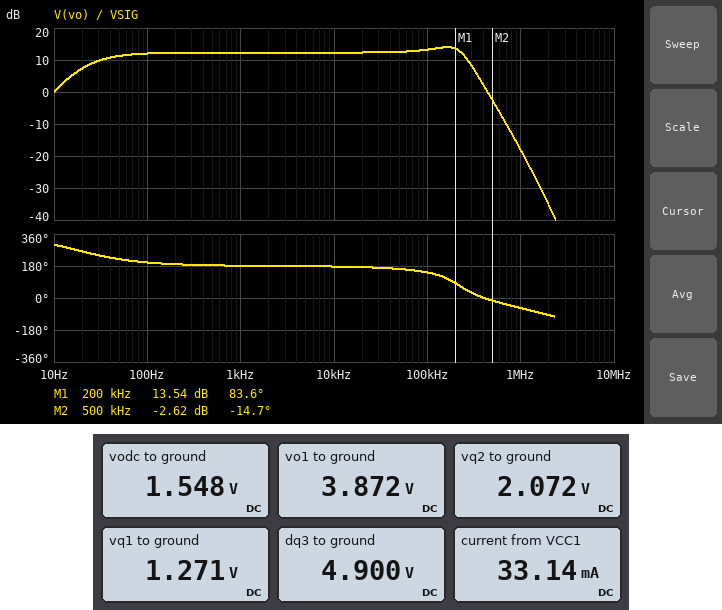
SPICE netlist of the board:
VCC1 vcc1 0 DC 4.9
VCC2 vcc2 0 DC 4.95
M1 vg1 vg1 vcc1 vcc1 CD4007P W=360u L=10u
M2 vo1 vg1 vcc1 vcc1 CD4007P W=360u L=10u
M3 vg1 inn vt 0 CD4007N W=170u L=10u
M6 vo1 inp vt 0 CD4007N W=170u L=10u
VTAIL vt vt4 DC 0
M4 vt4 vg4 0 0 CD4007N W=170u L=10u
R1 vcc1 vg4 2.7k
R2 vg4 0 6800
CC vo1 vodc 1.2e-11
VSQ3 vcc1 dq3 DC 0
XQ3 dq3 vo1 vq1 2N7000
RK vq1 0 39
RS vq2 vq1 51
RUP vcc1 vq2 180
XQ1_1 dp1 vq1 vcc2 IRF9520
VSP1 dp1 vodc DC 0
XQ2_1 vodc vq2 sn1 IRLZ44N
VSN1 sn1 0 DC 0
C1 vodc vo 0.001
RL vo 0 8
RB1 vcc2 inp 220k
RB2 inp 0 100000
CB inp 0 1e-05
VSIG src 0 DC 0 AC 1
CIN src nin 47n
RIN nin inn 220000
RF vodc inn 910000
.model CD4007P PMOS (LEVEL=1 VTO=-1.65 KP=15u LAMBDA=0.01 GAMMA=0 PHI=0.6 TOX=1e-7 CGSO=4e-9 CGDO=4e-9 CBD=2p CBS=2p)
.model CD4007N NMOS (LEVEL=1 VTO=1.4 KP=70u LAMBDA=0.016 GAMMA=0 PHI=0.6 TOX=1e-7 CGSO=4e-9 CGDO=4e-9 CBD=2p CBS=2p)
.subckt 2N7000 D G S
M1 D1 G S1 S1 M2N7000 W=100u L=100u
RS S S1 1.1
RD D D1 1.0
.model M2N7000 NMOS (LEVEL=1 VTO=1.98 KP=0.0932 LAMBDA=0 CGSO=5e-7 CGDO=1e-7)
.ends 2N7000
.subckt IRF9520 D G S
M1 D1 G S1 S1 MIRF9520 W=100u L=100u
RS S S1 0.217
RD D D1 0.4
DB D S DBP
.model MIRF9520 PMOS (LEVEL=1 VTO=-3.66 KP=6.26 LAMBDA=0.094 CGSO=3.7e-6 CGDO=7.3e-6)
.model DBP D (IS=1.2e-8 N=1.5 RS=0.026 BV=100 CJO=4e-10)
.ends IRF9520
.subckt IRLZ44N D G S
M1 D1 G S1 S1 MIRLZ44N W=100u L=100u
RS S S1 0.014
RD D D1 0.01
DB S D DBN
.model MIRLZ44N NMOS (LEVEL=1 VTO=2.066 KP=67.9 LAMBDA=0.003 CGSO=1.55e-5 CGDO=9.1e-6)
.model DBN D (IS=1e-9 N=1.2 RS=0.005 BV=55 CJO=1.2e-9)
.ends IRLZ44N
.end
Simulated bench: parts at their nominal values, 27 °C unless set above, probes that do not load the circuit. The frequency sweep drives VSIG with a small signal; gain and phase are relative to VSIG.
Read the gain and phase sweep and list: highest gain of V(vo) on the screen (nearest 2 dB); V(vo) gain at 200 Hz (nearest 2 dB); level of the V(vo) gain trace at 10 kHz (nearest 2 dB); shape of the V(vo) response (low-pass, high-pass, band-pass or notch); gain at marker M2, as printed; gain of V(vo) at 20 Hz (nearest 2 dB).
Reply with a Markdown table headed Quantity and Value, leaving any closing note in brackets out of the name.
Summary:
| Quantity | Value |
|---|---|
| highest gain of V(vo) on the screen | 14 dB |
| V(vo) gain at 200 Hz | 12 dB |
| level of the V(vo) gain trace at 10 kHz | 12 dB |
| shape of the V(vo) response | band-pass |
| gain at marker M2, as printed | -2.62 dB |
| gain of V(vo) at 20 Hz | 8 dB |
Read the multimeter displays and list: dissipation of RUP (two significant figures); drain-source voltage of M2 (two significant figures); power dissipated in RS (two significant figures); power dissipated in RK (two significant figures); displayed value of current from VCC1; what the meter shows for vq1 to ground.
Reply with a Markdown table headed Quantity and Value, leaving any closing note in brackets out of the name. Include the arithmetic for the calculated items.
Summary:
| Quantity | Value |
|---|---|
| dissipation of RUP | (4.9 V - 2.072 V)^2 / 180 Ω = 44 mW |
| drain-source voltage of M2 | 3.872 V - 4.9 V = -1.0 V |
| power dissipated in RS | (2.072 V - 1.271 V)^2 / 51 Ω = 13 mW |
| power dissipated in RK | (1.271 V)^2 / 39 Ω = 41 mW |
| displayed value of current from VCC1 | 33.14 mA |
| what the meter shows for vq1 to ground | 1.271 V |
